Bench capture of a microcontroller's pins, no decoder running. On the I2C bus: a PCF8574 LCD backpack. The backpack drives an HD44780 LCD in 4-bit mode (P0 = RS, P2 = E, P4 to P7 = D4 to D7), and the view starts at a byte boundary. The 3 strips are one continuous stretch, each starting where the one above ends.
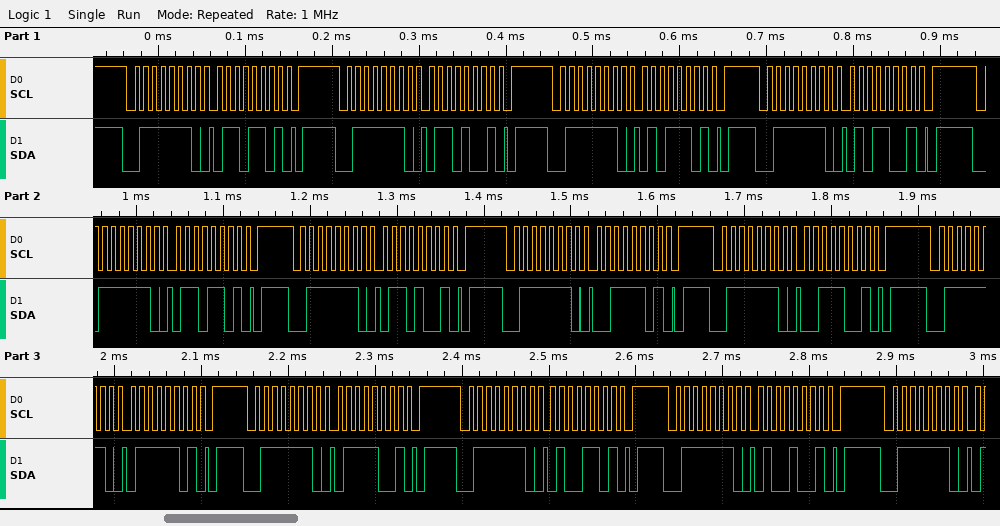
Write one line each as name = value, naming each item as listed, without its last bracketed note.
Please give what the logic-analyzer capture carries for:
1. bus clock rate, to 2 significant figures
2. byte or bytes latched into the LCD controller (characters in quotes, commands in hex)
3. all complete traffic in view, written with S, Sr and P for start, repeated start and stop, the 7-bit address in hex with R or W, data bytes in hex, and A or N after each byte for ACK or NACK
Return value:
bus clock rate, to 2 significant figures = 100 kHz
byte or bytes latched into the LCD controller = 'e' 'c' 't'
all complete traffic in view, written with S, Sr and P for start, repeated start and stop, the 7-bit address in hex with R or W, data bytes in hex, and A or N after each byte for ACK or NACK = S 3FW A 6D A P S 3FW A 69 A P S 3FW A 5D A P S 3FW A 59 A P S 3FW A 6D A P S 3FW A 69 A P S 3FW A 3D A P S 3FW A 39 A P S 3FW A 7D A P S 3FW A 79 A P S 3FW A 4D A P S 3FW A 49 A P S 3FW A
